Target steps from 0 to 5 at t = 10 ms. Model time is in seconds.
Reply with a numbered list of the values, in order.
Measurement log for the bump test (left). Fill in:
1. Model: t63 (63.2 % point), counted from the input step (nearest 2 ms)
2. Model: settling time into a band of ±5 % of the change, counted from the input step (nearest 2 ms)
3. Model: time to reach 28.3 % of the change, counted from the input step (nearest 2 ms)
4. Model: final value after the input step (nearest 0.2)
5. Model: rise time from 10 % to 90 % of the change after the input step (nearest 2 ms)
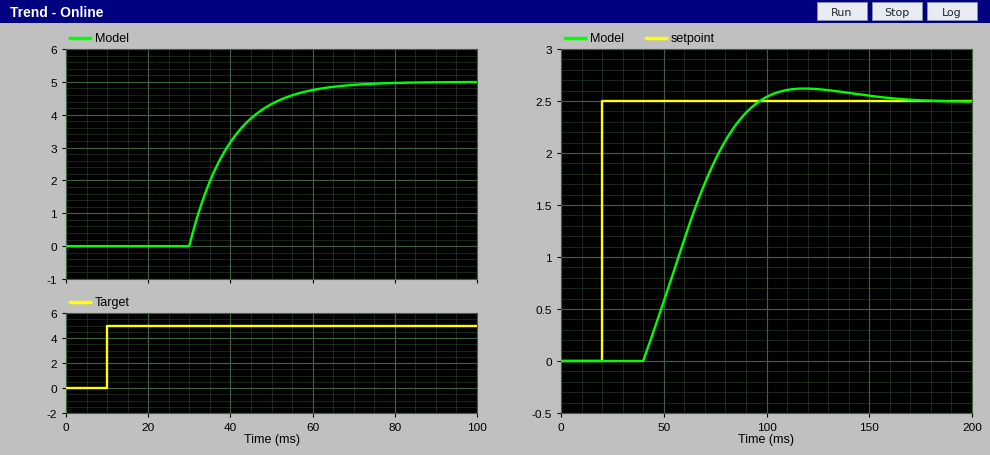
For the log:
1. 30 ms
2. 50 ms
3. 24 ms
4. 5.0
5. 22 ms
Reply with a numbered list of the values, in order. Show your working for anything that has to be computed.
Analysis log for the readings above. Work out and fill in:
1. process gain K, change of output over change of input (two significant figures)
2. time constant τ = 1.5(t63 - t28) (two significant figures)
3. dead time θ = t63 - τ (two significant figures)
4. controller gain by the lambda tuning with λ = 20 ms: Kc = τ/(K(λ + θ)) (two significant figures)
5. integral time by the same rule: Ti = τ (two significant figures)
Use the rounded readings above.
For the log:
1. (5 - 0) / 5 = 1.0
2. 1.5 × (30 - 24) = 9.0 ms
3. 30 - 9 = 21 ms
4. 9 / (1 × (20 + 21)) = 0.22
5. 9.0 ms
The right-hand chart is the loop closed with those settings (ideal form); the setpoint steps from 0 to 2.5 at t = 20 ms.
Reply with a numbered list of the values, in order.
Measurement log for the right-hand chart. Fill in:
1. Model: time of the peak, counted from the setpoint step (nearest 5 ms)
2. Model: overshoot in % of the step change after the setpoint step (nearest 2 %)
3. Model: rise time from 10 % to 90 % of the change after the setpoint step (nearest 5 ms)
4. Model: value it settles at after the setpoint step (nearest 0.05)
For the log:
1. 100 ms
2. 4 %
3. 40 ms
4. 2.50
